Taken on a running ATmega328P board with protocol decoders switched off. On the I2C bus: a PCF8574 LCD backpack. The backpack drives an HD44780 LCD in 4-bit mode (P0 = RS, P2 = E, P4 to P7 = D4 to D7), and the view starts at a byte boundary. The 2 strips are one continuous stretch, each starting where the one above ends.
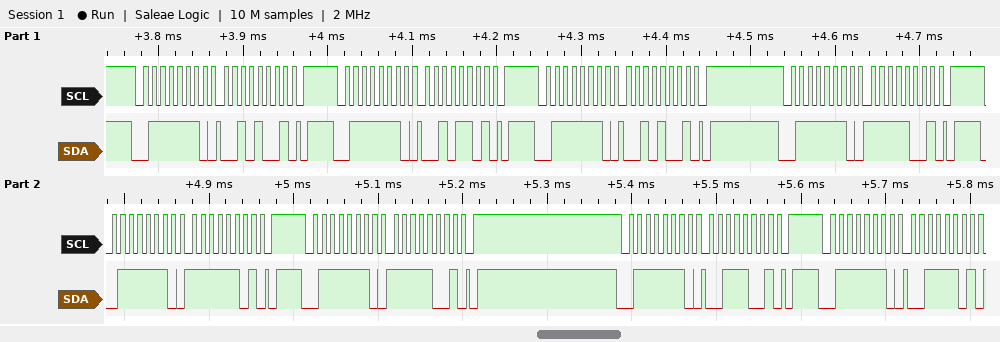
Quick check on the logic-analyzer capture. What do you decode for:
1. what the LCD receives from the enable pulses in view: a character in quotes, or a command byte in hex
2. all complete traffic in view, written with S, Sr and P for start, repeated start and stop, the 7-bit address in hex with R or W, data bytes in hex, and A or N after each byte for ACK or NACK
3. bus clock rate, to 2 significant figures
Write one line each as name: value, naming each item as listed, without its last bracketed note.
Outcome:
what the LCD receives from the enable pulses in view: a character in quotes, or a command byte in hex: '/'
all complete traffic in view, written with S, Sr and P for start, repeated start and stop, the 7-bit address in hex with R or W, data bytes in hex, and A or N after each byte for ACK or NACK: S 3FW A 29 A P S 3FW A 2D A P S 3FW A 29 A P S 3FW A F9 A P S 3FW A FD A P S 3FW A F9 A P S 3FW A 39 A P S 3FW A 3D A
bus clock rate, to 2 significant figures: 100 kHz
